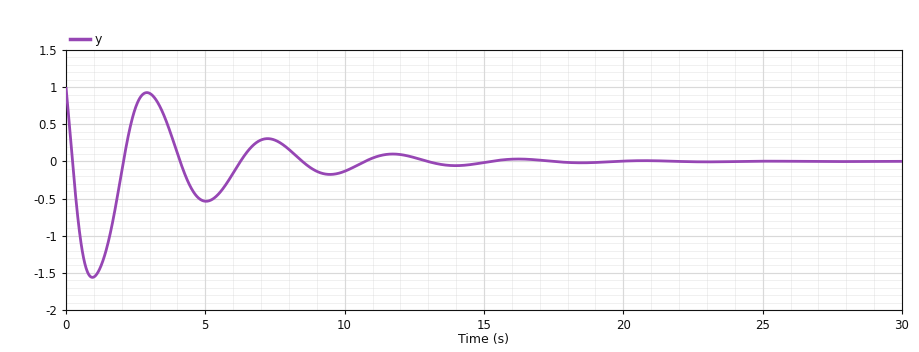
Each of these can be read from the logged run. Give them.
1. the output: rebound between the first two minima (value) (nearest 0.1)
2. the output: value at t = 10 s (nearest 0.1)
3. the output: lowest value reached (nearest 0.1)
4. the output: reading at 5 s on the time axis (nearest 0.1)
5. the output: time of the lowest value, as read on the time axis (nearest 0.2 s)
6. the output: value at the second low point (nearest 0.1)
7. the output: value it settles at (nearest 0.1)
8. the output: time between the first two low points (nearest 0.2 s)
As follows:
0.9
-0.1
-1.6
-0.5
1.0 s
-0.5
0.0
4.0 s
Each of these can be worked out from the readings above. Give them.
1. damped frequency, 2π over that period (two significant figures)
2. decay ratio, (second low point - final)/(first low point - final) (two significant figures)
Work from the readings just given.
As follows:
1.6 rad/s
0.31
